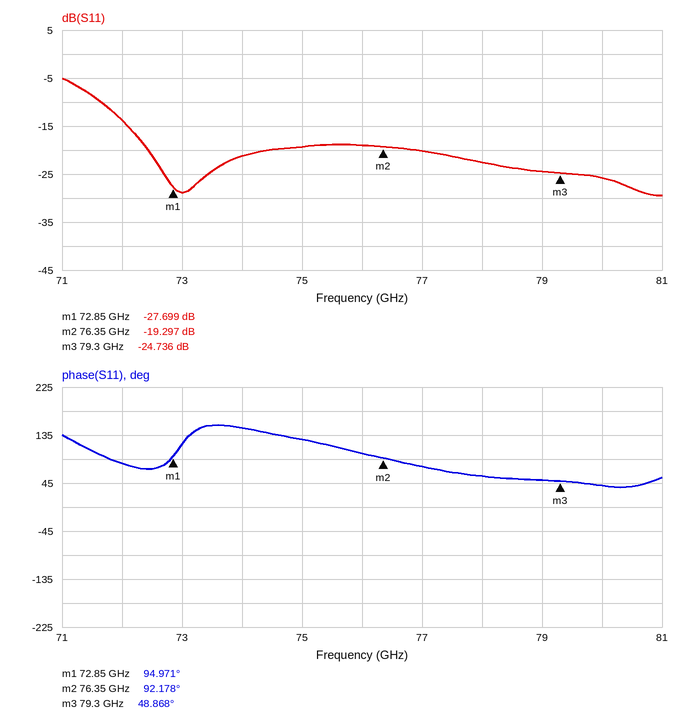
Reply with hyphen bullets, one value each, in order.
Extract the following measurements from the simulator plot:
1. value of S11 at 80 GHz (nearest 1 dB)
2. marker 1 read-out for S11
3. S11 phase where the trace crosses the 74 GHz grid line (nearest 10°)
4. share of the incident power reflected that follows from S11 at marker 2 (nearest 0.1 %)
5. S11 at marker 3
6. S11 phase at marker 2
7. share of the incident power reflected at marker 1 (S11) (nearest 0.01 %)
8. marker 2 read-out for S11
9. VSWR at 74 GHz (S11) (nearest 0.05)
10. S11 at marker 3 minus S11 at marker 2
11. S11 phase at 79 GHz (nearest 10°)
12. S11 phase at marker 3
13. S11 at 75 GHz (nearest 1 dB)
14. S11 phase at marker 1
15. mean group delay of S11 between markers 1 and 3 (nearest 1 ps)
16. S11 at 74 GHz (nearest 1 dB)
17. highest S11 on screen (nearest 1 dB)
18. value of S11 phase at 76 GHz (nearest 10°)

- -26 dB
- -27.699 dB
- 150°
- 1.2 %
- -24.736 dB
- 92.178°
- 0.17 %
- -19.297 dB
- 1.20
- -5.439 dB
- 50°
- 48.868°
- -19 dB
- 94.971°
- 20 ps
- -21 dB
- -5 dB
- 100°
